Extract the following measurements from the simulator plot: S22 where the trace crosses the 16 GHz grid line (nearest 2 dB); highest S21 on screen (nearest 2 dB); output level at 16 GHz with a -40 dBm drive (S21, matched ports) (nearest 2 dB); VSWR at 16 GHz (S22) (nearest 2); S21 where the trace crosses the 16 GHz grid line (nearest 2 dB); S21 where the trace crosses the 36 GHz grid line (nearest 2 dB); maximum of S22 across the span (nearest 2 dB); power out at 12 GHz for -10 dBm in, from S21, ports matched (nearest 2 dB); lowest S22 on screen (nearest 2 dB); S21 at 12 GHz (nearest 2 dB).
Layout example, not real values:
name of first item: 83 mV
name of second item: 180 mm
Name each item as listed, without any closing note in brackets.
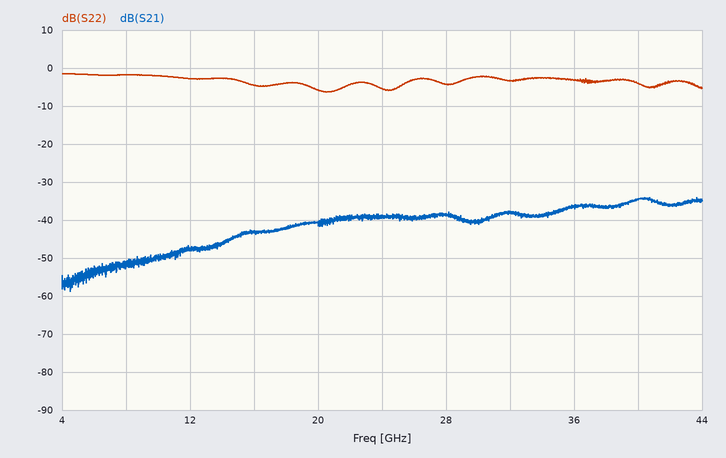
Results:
S22 where the trace crosses the 16 GHz grid line: -4 dB
highest S21 on screen: -34 dB
output level at 16 GHz with a -40 dBm drive (S21, matched ports): -84 dBm
VSWR at 16 GHz (S22): 4
S21 where the trace crosses the 16 GHz grid line: -44 dB
S21 where the trace crosses the 36 GHz grid line: -36 dB
maximum of S22 across the span: -2 dB
power out at 12 GHz for -10 dBm in, from S21, ports matched: -58 dBm
lowest S22 on screen: -6 dB
S21 at 12 GHz: -48 dB
